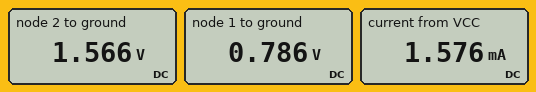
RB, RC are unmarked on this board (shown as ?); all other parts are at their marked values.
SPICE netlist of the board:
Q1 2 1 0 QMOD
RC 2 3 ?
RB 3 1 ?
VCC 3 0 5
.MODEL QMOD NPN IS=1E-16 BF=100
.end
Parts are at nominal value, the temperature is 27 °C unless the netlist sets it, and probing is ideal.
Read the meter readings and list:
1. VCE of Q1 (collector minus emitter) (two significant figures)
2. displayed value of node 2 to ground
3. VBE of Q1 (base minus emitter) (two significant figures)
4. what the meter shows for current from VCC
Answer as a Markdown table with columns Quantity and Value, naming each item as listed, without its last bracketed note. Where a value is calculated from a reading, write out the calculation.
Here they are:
| Quantity | Value |
|---|---|
| VCE of Q1 (collector minus emitter) | 1.566 V = 1.6 V |
| displayed value of node 2 to ground | 1.566 V |
| VBE of Q1 (base minus emitter) | 786 mV = 790 mV |
| what the meter shows for current from VCC | 1.576 mA |
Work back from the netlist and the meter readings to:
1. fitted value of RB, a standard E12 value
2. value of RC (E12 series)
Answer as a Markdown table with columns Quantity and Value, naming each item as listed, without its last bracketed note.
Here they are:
| Quantity | Value |
|---|---|
| fitted value of RB, a standard E12 value | 270 kΩ |
| value of RC | 2.2 kΩ |
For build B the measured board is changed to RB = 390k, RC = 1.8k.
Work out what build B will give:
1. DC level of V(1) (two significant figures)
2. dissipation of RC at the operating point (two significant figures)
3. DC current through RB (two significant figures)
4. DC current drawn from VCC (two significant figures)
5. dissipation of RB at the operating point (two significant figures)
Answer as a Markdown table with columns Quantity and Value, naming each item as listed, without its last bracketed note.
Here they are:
| Quantity | Value |
|---|---|
| DC level of V(1) | 780 mV |
| dissipation of RC at the operating point | 2.1 mW |
| DC current through RB | 11 µA |
| DC current drawn from VCC | 1.1 mA |
| dissipation of RB at the operating point | 46 µW |
